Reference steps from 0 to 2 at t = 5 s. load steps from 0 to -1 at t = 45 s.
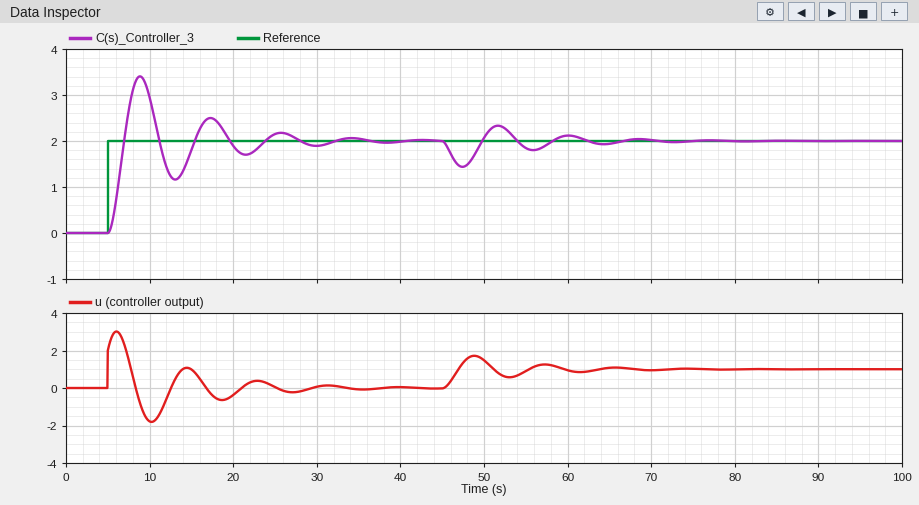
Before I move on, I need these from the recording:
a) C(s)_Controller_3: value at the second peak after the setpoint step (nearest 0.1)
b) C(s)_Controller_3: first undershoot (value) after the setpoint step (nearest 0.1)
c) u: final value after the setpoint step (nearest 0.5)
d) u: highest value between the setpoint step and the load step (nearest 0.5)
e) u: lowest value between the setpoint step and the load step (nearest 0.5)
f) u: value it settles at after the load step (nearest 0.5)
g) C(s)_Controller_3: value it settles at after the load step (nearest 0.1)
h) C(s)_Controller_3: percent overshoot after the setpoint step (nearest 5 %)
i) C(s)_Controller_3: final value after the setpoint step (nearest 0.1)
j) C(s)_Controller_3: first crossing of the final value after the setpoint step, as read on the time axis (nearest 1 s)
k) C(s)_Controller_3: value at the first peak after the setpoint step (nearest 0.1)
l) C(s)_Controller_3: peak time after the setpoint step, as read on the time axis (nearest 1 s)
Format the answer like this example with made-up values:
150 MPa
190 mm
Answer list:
2.5
1.2
0.0
3.0
-2.0
1.0
2.0
70 %
2.0
7 s
3.4
9 s
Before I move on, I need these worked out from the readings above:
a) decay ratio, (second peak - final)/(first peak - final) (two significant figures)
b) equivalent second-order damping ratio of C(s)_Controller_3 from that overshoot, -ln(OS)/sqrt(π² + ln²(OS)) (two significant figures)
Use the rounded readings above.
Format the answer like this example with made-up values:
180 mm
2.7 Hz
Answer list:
0.36
0.11
